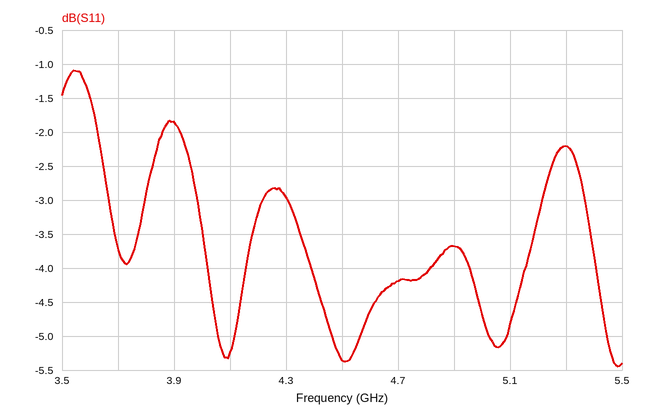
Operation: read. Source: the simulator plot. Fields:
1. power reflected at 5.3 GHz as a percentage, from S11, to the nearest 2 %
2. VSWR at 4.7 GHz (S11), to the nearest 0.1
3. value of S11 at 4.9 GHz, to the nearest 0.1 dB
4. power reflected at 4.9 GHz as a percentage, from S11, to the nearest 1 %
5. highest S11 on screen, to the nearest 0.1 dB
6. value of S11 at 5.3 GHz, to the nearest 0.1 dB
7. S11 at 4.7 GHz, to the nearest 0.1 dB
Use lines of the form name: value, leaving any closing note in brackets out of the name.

power reflected at 5.3 GHz as a percentage, from S11, to the nearest 2 %: 60 %
VSWR at 4.7 GHz (S11), to the nearest 0.1: 4.2
value of S11 at 4.9 GHz, to the nearest 0.1 dB: -3.7 dB
power reflected at 4.9 GHz as a percentage, from S11, to the nearest 1 %: 43 %
highest S11 on screen, to the nearest 0.1 dB: -1.1 dB
value of S11 at 5.3 GHz, to the nearest 0.1 dB: -2.2 dB
S11 at 4.7 GHz, to the nearest 0.1 dB: -4.2 dB
